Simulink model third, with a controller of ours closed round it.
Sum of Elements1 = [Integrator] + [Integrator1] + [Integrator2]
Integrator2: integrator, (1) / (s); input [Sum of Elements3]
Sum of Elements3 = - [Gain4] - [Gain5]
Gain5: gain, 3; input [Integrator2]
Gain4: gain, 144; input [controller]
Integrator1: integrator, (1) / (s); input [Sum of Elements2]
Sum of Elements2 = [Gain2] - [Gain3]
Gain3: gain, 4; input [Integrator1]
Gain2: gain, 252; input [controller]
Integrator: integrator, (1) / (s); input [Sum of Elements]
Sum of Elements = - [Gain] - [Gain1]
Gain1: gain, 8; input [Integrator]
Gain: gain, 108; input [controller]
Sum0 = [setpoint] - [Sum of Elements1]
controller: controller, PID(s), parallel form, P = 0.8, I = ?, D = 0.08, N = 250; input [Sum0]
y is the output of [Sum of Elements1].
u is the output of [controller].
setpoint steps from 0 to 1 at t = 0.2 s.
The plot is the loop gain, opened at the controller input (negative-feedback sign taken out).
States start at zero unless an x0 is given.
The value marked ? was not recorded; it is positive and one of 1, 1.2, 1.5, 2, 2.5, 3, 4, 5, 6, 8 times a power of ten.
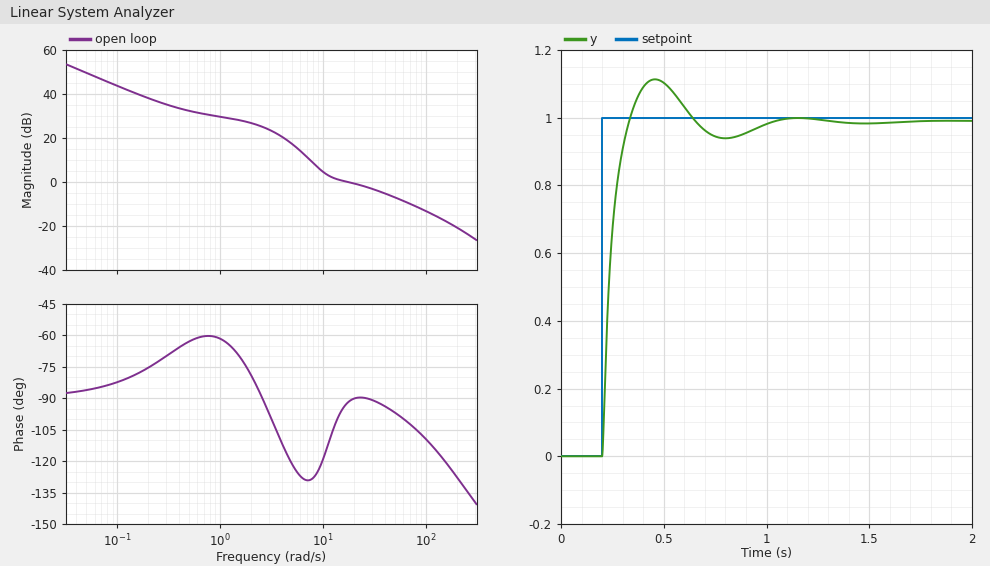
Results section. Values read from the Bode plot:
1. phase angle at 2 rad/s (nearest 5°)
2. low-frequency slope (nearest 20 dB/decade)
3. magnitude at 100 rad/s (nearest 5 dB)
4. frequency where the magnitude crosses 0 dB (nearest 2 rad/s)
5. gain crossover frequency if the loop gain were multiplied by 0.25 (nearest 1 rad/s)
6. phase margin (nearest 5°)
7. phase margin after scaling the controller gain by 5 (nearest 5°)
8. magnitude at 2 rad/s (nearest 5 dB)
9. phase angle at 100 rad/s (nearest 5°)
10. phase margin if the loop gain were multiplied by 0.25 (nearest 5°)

-80°
-20 dB/decade
-15 dB
18 rad/s
7 rad/s
90°
70°
25 dB
-110°
50°
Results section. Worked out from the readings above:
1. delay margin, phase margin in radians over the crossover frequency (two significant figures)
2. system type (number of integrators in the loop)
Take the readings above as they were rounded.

0.087 s
1
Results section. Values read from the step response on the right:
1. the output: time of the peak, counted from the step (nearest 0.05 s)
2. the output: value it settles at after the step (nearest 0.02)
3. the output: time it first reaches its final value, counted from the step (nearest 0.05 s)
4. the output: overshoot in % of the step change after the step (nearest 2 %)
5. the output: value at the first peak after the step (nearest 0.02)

0.25 s
1.00
0.15 s
12 %
1.12
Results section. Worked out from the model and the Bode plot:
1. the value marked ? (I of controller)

10
